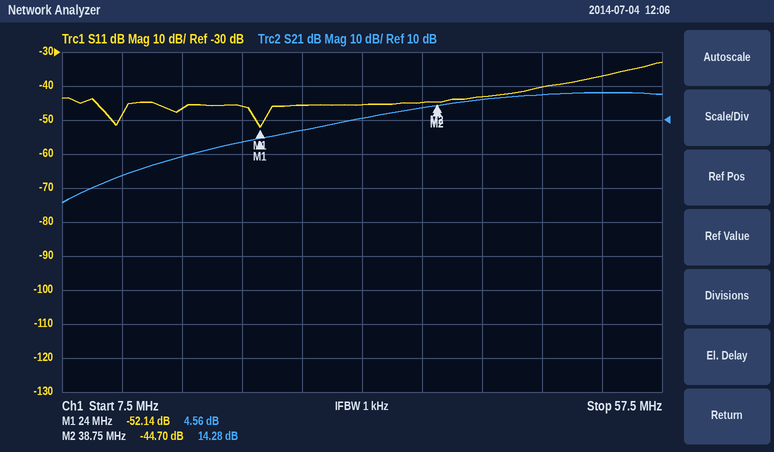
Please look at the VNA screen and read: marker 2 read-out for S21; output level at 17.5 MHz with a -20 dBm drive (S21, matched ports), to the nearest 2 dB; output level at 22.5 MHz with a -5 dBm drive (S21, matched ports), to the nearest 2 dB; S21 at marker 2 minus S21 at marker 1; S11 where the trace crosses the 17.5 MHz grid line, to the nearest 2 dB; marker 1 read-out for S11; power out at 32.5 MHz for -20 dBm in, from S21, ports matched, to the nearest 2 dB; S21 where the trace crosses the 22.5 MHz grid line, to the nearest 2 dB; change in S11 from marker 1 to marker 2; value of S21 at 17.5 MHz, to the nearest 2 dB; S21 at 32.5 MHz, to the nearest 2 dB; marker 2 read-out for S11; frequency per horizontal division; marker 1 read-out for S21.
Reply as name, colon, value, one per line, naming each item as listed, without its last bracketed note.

marker 2 read-out for S21: 14.28 dB
output level at 17.5 MHz with a -20 dBm drive (S21, matched ports), to the nearest 2 dB: -20 dBm
output level at 22.5 MHz with a -5 dBm drive (S21, matched ports), to the nearest 2 dB: -2 dBm
S21 at marker 2 minus S21 at marker 1: 9.72 dB
S11 where the trace crosses the 17.5 MHz grid line, to the nearest 2 dB: -46 dB
marker 1 read-out for S11: -52.14 dB
power out at 32.5 MHz for -20 dBm in, from S21, ports matched, to the nearest 2 dB: -10 dBm
S21 where the trace crosses the 22.5 MHz grid line, to the nearest 2 dB: 4 dB
change in S11 from marker 1 to marker 2: 7.44 dB
value of S21 at 17.5 MHz, to the nearest 2 dB: 0 dB
S21 at 32.5 MHz, to the nearest 2 dB: 10 dB
marker 2 read-out for S11: -44.70 dB
frequency per horizontal division: 5 MHz
marker 1 read-out for S21: 4.56 dB
